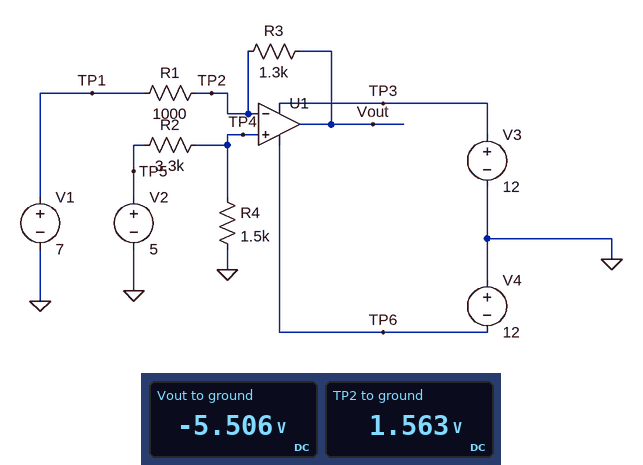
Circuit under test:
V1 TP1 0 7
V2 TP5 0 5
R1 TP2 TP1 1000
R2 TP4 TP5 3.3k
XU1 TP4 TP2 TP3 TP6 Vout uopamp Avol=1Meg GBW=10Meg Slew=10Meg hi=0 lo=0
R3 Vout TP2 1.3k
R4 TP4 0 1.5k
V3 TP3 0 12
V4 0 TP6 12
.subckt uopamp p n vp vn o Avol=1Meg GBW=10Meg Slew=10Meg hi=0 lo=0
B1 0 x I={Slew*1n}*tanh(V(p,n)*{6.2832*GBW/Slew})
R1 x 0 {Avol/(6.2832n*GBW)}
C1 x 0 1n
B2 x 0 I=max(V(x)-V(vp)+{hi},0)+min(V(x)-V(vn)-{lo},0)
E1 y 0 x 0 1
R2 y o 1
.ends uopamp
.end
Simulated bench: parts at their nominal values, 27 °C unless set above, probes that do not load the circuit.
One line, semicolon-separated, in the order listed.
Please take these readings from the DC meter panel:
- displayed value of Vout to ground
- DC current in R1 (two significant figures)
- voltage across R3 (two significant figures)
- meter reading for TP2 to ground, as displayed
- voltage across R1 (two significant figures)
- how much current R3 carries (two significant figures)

-5.506 V; 5.4 mA; 7.1 V; 1.563 V; 5.4 V; 5.4 mA
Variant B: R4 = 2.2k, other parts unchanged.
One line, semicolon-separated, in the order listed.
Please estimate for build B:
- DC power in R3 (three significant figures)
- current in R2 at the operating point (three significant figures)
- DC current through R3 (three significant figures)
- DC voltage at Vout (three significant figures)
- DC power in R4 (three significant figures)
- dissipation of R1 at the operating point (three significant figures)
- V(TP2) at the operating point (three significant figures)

32.5 mW; 909 µA; 5.00 mA; -4.50 V; 1.82 mW; 25.0 mW; 2.00 V
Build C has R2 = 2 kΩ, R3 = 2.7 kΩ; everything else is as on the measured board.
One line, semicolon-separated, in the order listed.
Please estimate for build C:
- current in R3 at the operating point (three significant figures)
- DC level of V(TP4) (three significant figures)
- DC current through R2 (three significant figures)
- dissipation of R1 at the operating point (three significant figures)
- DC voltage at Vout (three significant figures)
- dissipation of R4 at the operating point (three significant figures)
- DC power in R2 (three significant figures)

4.86 mA; 2.14 V; 1.43 mA; 23.6 mW; -11.0 V; 3.06 mW; 4.08 mW
